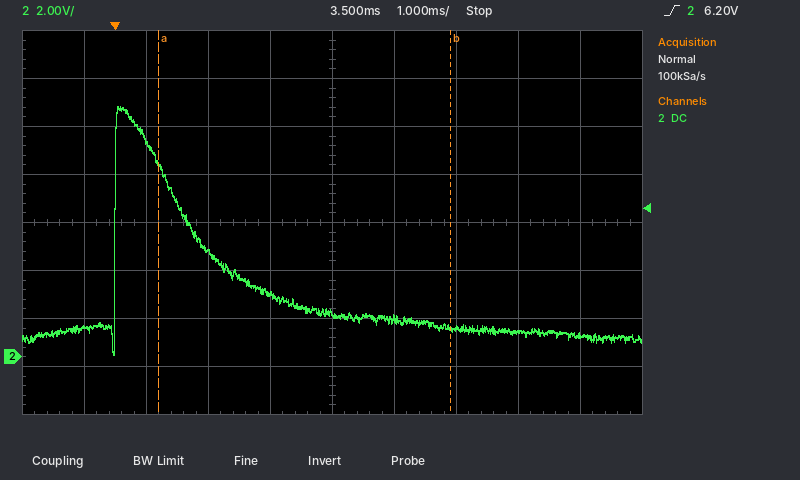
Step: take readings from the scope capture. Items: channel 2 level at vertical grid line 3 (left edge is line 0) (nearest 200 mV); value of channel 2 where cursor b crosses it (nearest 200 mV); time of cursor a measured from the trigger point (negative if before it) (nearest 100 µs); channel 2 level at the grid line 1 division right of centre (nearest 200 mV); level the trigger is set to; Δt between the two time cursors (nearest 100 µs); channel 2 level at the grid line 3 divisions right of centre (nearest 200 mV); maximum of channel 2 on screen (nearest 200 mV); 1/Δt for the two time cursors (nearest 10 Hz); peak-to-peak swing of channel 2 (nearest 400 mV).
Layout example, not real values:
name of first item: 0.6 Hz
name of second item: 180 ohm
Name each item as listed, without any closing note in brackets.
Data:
channel 2 level at vertical grid line 3 (left edge is line 0): 4.4 V
value of channel 2 where cursor b crosses it: 1.2 V
time of cursor a measured from the trigger point (negative if before it): +700 µs
channel 2 level at the grid line 1 division right of centre: 1.6 V
level the trigger is set to: 6.20 V
Δt between the two time cursors: 4.7 ms
channel 2 level at the grid line 3 divisions right of centre: 1.0 V
maximum of channel 2 on screen: 10.4 V
1/Δt for the two time cursors: 210 Hz
peak-to-peak swing of channel 2: 10.4 V
